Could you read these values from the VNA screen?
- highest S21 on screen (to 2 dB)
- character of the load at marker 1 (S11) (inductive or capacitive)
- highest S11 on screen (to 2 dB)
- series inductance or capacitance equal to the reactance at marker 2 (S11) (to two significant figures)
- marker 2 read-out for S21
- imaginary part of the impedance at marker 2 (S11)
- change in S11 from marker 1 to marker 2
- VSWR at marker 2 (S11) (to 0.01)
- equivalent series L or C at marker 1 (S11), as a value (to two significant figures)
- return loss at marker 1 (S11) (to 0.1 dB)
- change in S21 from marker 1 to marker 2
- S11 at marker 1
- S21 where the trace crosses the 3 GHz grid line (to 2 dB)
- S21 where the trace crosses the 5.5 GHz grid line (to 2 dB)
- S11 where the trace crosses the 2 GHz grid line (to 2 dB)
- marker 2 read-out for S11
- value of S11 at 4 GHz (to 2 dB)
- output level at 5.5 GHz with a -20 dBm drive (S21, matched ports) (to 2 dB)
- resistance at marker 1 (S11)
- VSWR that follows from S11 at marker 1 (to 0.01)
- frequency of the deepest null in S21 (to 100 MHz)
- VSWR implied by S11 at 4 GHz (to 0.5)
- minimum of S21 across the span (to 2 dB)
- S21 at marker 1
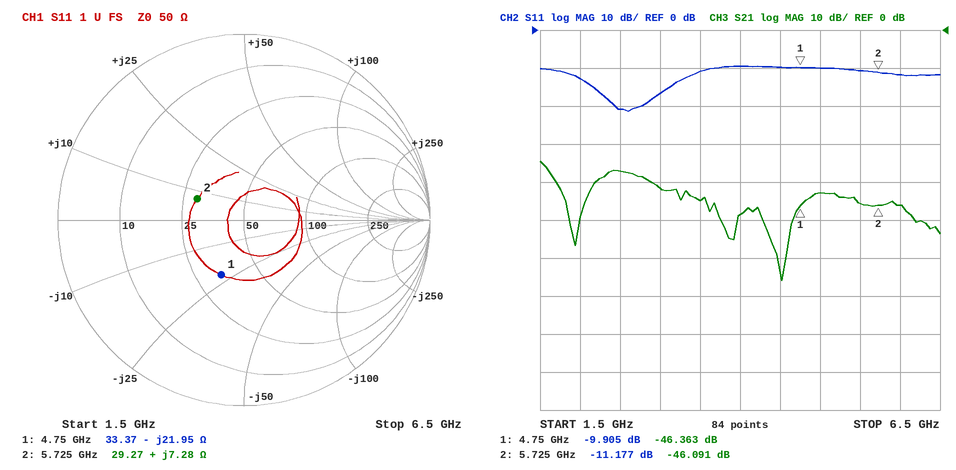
-34 dB
capacitive
-10 dB
200 pH
-46.091 dB
+7.28 Ω
-1.272 dB
1.76
1.5 pF
9.9 dB
0.272 dB
-9.905 dB
-42 dB
-46 dB
-12 dB
-11.177 dB
-10 dB
-66 dBm
33.37 Ω
1.94
4.5 GHz
2.0
-66 dB
-46.363 dB
